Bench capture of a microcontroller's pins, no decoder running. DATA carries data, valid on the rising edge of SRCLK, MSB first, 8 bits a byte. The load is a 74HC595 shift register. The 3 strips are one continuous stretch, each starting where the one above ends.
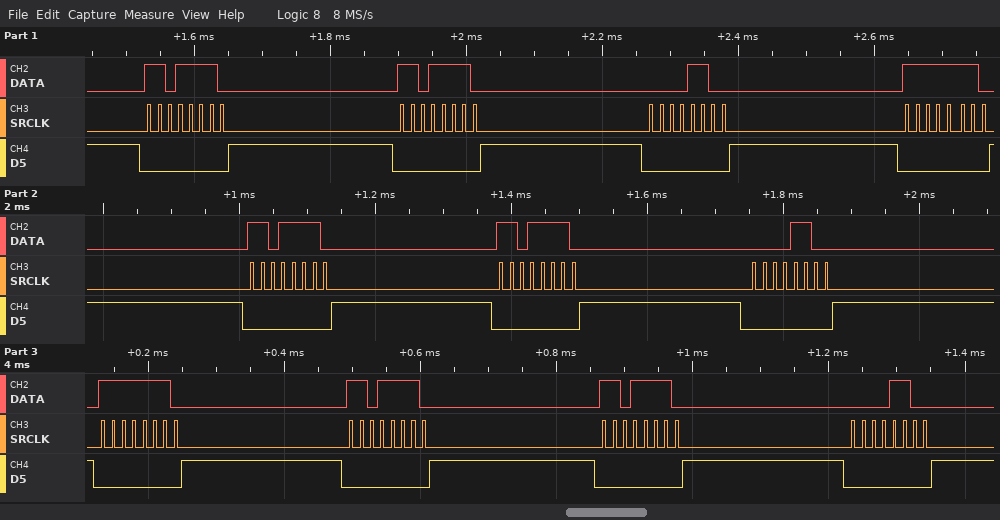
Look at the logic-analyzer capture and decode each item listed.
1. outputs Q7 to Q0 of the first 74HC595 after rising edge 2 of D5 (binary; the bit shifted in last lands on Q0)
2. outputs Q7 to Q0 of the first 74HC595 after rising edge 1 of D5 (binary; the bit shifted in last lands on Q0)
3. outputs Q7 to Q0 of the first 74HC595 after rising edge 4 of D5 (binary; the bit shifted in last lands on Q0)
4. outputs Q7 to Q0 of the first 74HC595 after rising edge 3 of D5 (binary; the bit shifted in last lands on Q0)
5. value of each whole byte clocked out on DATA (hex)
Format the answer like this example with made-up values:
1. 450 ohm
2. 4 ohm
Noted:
1. 11011110
2. 11011110
3. 11111110
4. 00001100
5. DE DE 0C FE DE DE 0C FE DE DE 0C
